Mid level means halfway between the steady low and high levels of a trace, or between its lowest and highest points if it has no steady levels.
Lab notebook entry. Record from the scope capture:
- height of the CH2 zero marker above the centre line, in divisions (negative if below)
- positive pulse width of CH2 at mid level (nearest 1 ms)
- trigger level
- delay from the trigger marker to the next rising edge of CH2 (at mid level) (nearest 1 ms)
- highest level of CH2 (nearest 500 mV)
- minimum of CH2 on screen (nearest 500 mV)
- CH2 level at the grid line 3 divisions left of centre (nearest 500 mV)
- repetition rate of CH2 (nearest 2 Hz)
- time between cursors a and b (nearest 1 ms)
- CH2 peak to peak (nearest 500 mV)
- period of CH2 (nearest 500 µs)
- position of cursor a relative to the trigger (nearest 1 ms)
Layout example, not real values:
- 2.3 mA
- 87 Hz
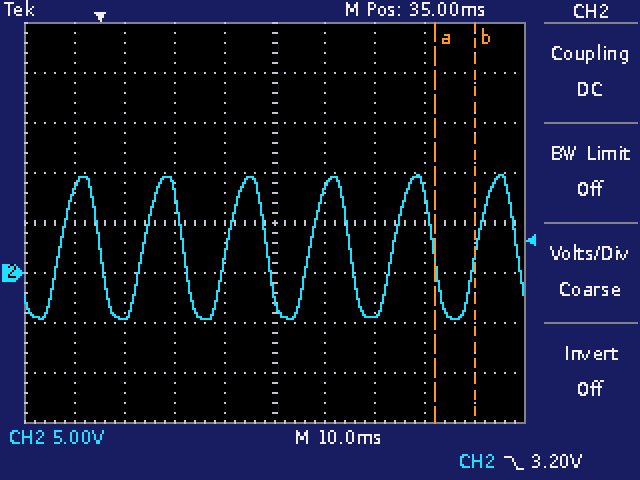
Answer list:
- -1.0 div
- 8 ms
- 3.20 V
- 9 ms
- 10.0 V
- -4.5 V
- -4.5 V
- 60 Hz
- 8 ms
- 14.5 V
- 16.5 ms
- +67 ms
